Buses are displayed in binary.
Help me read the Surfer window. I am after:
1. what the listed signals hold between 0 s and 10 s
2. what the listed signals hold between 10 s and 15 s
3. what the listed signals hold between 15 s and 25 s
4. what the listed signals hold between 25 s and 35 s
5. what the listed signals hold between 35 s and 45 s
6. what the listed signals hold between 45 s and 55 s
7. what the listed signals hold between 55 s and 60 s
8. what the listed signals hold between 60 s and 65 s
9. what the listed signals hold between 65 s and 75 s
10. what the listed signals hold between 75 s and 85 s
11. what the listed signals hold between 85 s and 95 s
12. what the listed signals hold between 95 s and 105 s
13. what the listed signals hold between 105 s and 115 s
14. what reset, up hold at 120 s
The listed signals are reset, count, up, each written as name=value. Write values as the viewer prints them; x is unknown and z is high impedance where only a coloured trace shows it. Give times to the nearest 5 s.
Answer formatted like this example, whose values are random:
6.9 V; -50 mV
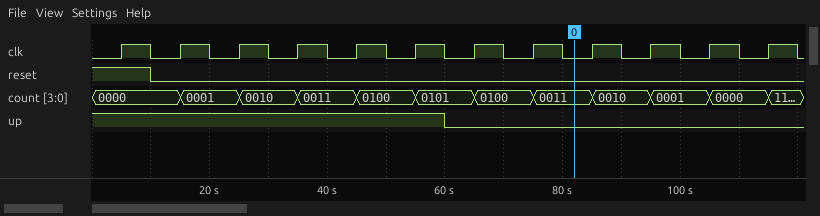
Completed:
reset=1, count=0000, up=1; reset=0, count=0000, up=1; reset=0, count=0001, up=1; reset=0, count=0010, up=1; reset=0, count=0011, up=1; reset=0, count=0100, up=1; reset=0, count=0101, up=1; reset=0, count=0101, up=0; reset=0, count=0100, up=0; reset=0, count=0011, up=0; reset=0, count=0010, up=0; reset=0, count=0001, up=0; reset=0, count=0000, up=0; reset=0, up=0
